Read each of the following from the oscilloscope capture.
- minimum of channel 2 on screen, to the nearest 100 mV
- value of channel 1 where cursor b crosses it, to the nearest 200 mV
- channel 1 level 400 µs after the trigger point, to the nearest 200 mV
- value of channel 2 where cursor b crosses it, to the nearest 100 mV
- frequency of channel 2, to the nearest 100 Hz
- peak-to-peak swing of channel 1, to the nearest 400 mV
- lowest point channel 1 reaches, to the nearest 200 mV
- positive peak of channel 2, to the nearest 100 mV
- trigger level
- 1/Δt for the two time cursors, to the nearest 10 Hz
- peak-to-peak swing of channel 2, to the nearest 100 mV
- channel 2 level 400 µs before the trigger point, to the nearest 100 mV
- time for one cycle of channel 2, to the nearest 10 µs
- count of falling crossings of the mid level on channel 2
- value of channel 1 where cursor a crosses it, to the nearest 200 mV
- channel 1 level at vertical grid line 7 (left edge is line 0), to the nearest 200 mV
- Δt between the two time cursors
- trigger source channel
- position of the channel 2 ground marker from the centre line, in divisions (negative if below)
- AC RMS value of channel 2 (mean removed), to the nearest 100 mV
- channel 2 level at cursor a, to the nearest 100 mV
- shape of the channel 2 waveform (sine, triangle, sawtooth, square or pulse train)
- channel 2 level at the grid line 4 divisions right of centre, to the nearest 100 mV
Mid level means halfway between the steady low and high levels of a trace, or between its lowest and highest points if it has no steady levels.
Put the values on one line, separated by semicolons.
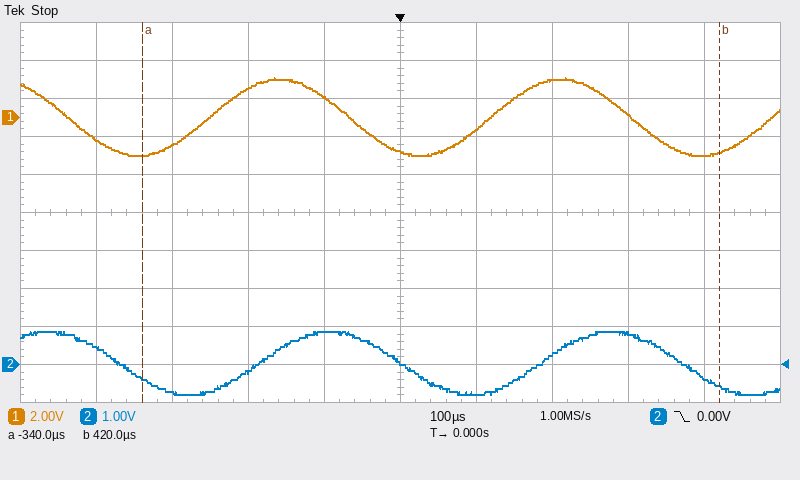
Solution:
-800 mV; -1.8 V; -2.0 V; -600 mV; 2.7 kHz; 4.0 V; -2.0 V; 900 mV; 0.00 V; 1.32 kHz; 1.7 V; 500 mV; 370 µs; 3; -2.0 V; 2.0 V; 760 µs; channel 2; -4.0 div; 600 mV; -400 mV; sine; -400 mV
